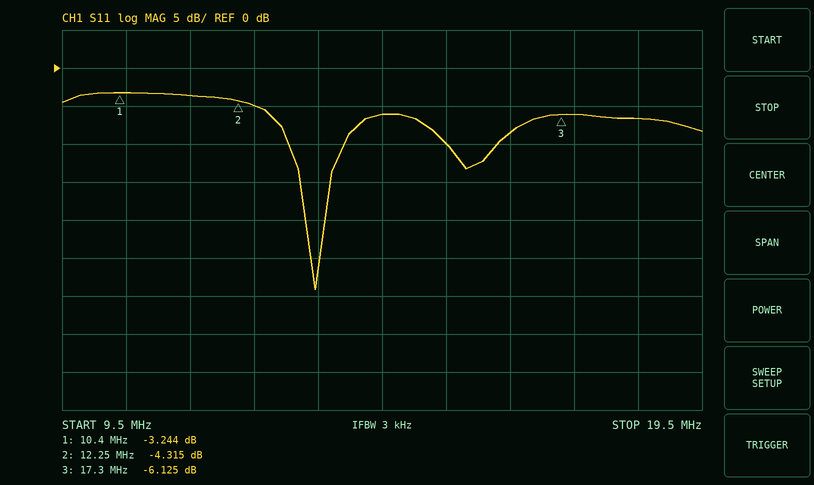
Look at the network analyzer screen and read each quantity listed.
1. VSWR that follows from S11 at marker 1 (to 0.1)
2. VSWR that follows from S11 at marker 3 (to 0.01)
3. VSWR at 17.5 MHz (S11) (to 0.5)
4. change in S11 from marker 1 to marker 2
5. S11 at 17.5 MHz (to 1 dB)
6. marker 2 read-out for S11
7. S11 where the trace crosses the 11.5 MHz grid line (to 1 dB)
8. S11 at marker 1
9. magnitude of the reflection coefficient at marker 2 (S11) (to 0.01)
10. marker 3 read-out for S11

5.4
2.95
3.0
-1.071 dB
-6 dB
-4.315 dB
-4 dB
-3.244 dB
0.61
-6.125 dB
